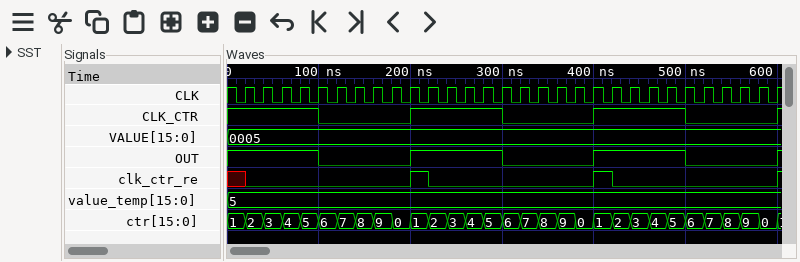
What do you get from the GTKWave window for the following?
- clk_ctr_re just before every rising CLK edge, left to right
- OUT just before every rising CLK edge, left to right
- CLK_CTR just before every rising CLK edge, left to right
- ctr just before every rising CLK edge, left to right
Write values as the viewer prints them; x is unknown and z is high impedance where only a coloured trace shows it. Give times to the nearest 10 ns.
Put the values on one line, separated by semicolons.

x 0 0 0 0 0 0 0 0 0 1 0 0 0 0 0 0 0 0 0 1 0 0 0 0 0 0 0 0 0; 1 1 1 1 1 0 0 0 0 0 1 1 1 1 1 0 0 0 0 0 1 1 1 1 1 0 0 0 0 0; 1 1 1 1 1 0 0 0 0 0 1 1 1 1 1 0 0 0 0 0 1 1 1 1 1 0 0 0 0 0; 1, 2, 3, 4, 5, 6, 7, 8, 9, 0, 1, 2, 3, 4, 5, 6, 7, 8, 9, 0, 1, 2, 3, 4, 5, 6, 7, 8, 9, 0
